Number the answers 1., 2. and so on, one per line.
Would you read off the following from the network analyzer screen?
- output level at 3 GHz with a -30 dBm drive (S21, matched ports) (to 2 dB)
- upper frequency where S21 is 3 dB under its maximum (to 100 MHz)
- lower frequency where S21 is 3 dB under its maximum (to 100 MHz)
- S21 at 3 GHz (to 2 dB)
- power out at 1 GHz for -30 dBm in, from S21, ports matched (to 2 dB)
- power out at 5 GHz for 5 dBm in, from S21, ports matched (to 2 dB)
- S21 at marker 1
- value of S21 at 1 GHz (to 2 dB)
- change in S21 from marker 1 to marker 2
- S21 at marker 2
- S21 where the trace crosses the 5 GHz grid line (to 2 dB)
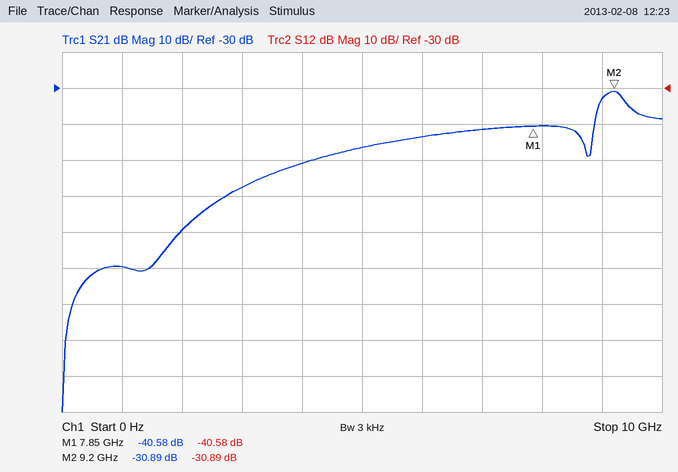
1. -88 dBm
2. 9.4 GHz
3. 9.0 GHz
4. -58 dB
5. -110 dBm
6. -42 dBm
7. -40.58 dB
8. -80 dB
9. 9.69 dB
10. -30.89 dB
11. -46 dB
